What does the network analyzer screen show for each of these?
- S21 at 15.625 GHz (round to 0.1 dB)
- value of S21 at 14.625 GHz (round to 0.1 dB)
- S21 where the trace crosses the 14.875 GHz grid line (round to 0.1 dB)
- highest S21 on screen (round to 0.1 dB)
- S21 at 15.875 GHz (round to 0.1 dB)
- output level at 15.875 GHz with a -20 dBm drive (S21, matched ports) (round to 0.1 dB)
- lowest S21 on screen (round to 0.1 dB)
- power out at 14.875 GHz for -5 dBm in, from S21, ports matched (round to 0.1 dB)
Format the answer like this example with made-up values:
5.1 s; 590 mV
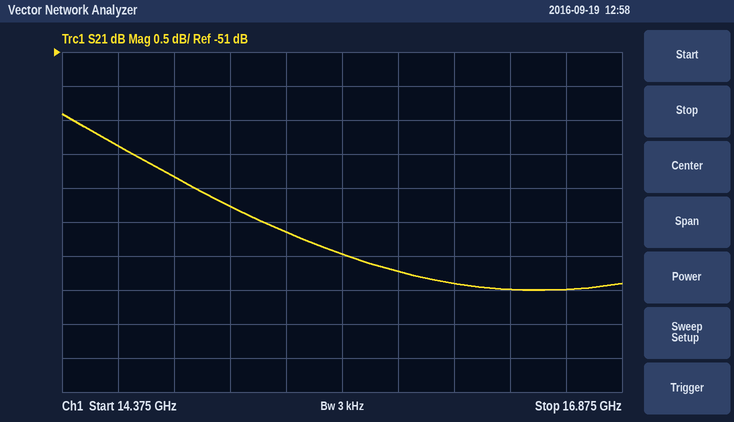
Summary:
-54.0 dB; -52.4 dB; -52.8 dB; -51.9 dB; -54.2 dB; -74.2 dBm; -54.5 dB; -57.8 dBm
